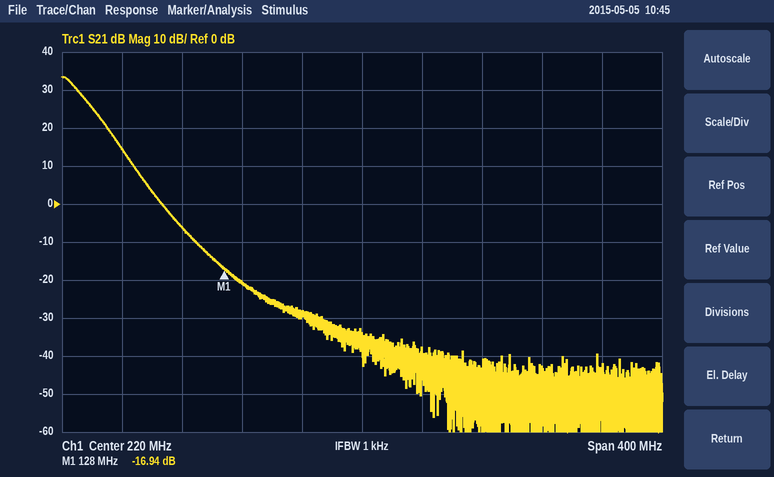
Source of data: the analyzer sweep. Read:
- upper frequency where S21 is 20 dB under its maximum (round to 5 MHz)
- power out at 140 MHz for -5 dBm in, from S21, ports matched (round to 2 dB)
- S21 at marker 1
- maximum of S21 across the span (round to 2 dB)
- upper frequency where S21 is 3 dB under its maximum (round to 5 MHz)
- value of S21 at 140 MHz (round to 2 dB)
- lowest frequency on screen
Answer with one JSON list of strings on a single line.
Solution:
["60 MHz", "-26 dBm", "-16.94 dB", "34 dB", "30 MHz", "-20 dB", "20 MHz"]
